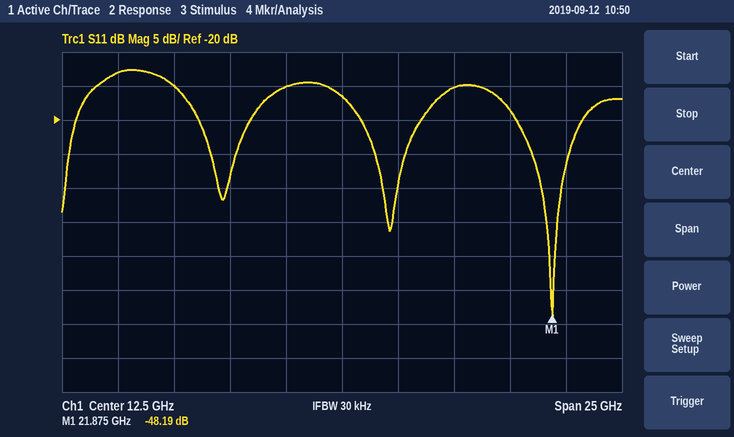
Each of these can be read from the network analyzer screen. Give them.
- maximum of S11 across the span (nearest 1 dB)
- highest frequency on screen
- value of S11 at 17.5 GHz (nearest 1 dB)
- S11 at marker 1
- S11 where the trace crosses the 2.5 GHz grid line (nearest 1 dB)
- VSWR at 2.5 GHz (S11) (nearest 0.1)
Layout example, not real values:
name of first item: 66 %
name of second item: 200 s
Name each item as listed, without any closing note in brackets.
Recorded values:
maximum of S11 across the span: -13 dB
highest frequency on screen: 25 GHz
value of S11 at 17.5 GHz: -15 dB
S11 at marker 1: -48.19 dB
S11 where the trace crosses the 2.5 GHz grid line: -13 dB
VSWR at 2.5 GHz (S11): 1.6
